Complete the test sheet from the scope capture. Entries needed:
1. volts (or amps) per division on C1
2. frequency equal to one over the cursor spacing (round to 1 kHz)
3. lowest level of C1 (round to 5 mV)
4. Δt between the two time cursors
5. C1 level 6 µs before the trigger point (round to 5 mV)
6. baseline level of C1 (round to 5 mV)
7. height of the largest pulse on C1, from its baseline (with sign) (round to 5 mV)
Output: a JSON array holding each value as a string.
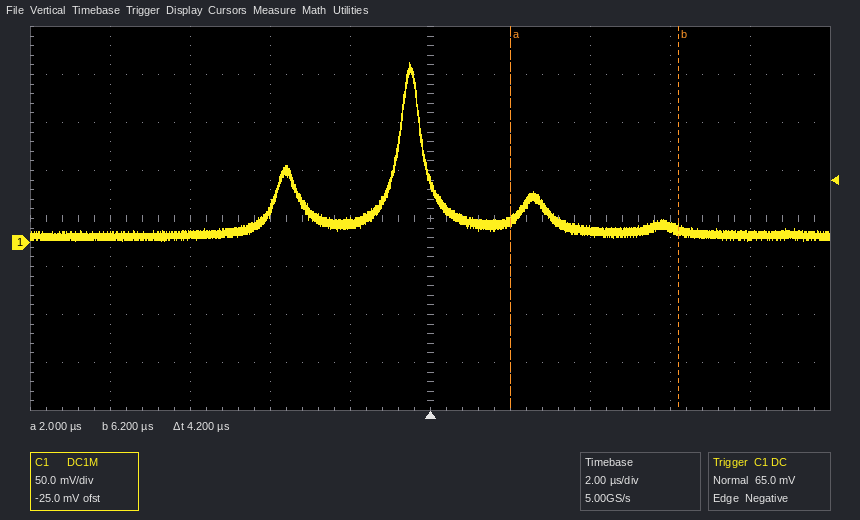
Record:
["50 mV", "238 kHz", "0 mV", "4.2 µs", "10 mV", "10 mV", "+180 mV"]
